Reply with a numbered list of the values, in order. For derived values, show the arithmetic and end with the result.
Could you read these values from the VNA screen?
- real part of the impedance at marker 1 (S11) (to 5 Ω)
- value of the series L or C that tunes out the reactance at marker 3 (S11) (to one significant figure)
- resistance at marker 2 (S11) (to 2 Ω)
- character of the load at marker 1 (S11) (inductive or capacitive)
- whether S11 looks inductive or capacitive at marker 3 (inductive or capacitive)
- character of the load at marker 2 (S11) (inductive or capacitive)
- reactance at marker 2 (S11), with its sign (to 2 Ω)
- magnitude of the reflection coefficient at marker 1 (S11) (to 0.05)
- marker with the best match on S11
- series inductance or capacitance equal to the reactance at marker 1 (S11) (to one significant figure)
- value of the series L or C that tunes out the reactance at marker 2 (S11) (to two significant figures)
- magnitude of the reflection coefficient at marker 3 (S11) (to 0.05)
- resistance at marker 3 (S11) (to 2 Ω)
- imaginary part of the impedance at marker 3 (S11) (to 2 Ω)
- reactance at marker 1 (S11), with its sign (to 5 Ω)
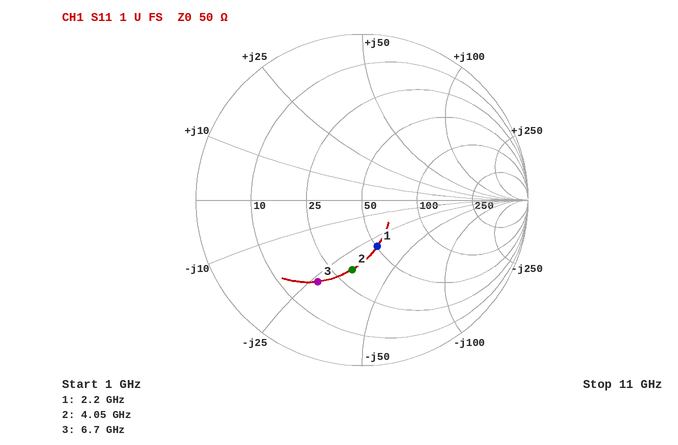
1. 50 Ω
2. L = 26 Ω/(2π × 6.7 GHz) ≈ 618 pH, so 600 pH to one significant figure
3. 32 Ω
4. capacitive
5. capacitive
6. capacitive
7. -32 Ω
8. 0.30
9. marker 1
10. C = 1/(2π × 2.2 GHz × 30 Ω) ≈ 2 pF
11. L = 32 Ω/(2π × 4.05 GHz) ≈ 1.3 nH
12. 0.55
13. 18 Ω
14. -26 Ω
15. -30 Ω
